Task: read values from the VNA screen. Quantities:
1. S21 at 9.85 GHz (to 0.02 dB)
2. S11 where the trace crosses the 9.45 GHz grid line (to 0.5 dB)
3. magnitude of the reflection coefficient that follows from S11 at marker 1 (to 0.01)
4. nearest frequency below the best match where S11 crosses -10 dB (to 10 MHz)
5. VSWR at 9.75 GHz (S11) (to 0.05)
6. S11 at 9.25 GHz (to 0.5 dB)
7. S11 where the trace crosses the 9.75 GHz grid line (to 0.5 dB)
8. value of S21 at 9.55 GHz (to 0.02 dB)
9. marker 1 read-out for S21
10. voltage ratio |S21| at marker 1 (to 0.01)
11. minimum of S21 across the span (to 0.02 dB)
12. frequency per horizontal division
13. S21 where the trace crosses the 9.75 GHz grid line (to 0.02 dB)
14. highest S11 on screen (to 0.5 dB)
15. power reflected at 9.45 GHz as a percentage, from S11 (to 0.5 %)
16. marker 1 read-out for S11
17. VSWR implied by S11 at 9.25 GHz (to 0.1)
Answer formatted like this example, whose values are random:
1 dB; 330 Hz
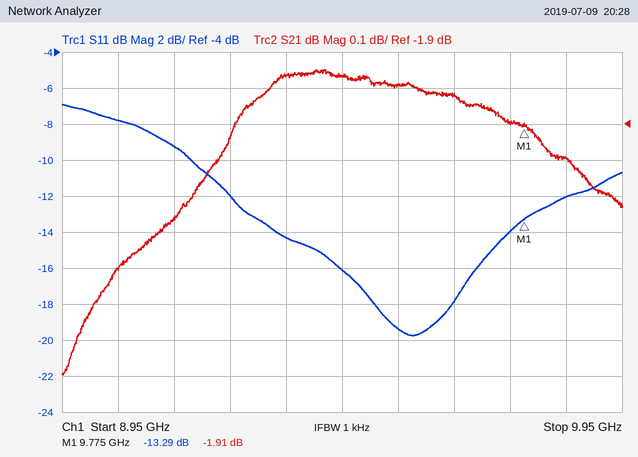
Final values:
-2.00 dB; -16.0 dB; 0.22; 9.18 GHz; 1.50; -12.0 dB; -14.0 dB; -1.80 dB; -1.91 dB; 0.80; -2.60 dB; 100 MHz; -1.90 dB; -7.0 dB; 2.5 %; -13.29 dB; 1.7
